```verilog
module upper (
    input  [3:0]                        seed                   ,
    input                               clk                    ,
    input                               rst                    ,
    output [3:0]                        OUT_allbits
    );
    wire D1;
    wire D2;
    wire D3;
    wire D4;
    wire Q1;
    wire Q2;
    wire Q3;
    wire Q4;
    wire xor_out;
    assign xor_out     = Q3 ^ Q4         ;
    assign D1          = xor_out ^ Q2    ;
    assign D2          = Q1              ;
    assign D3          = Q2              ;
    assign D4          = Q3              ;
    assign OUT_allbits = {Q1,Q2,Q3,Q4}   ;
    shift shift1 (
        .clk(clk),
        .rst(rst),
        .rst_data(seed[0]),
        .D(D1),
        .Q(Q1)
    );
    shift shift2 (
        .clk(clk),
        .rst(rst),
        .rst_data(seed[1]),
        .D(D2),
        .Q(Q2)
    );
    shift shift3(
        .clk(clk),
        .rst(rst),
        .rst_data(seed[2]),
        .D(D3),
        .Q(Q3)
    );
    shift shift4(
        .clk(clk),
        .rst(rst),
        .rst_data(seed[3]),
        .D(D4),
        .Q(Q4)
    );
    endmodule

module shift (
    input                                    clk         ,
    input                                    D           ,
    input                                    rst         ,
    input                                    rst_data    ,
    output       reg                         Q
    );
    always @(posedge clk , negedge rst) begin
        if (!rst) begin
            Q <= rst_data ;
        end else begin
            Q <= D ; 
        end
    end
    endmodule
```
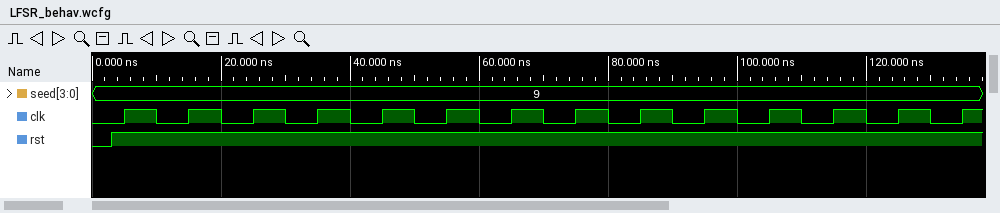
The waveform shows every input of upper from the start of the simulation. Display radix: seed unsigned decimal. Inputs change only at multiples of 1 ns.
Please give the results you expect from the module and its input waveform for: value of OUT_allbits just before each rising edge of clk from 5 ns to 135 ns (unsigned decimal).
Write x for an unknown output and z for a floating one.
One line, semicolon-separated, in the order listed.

9, 12, 14, 7, 11, 5, 2, 9, 12, 14, 7, 11, 5, 2
